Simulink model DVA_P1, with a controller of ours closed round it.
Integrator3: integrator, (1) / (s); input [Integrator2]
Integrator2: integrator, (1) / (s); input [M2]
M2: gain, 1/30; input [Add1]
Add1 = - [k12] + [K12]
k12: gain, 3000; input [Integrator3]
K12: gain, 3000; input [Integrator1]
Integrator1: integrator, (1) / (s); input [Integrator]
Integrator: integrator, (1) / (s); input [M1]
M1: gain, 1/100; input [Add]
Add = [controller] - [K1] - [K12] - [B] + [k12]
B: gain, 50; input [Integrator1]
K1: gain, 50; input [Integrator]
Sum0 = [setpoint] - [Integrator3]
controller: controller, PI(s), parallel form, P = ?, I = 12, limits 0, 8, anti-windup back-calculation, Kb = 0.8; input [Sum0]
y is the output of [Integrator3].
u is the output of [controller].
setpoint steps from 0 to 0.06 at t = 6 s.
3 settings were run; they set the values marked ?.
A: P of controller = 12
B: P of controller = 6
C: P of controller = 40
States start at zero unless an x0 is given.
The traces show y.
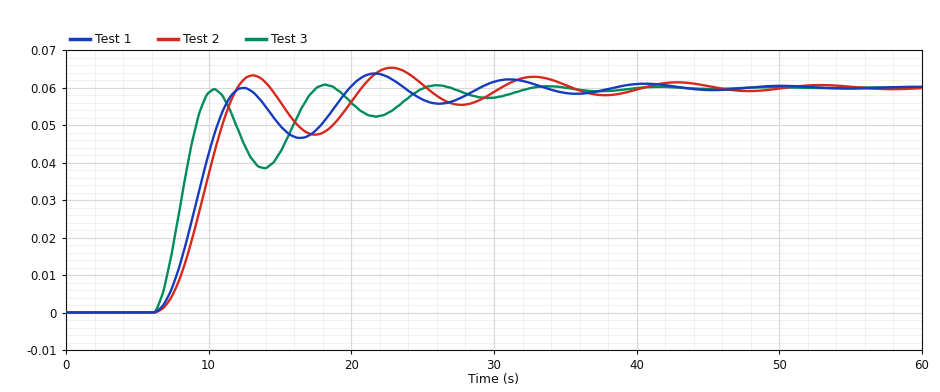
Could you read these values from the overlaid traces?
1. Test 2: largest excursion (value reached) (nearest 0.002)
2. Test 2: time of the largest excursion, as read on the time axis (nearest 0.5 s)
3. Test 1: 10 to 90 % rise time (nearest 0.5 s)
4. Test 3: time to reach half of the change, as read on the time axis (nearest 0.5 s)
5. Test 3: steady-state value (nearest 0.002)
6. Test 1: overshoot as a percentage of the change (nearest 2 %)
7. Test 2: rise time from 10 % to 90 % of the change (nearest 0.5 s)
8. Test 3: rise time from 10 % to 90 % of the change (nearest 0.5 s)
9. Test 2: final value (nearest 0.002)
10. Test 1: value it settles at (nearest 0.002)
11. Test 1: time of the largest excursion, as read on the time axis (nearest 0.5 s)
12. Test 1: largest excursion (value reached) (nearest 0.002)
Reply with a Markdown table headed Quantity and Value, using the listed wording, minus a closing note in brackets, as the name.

| Quantity | Value |
|---|---|
| Test 2: largest excursion (value reached) | 0.066 |
| Test 2: time of the largest excursion, as read on the time axis | 23.0 s |
| Test 1: 10 to 90 % rise time | 3.5 s |
| Test 3: time to reach half of the change, as read on the time axis | 8.0 s |
| Test 3: steady-state value | 0.060 |
| Test 1: overshoot as a percentage of the change | 6 % |
| Test 2: rise time from 10 % to 90 % of the change | 3.5 s |
| Test 3: rise time from 10 % to 90 % of the change | 2.5 s |
| Test 2: final value | 0.060 |
| Test 1: value it settles at | 0.060 |
| Test 1: time of the largest excursion, as read on the time axis | 21.5 s |
| Test 1: largest excursion (value reached) | 0.064 |
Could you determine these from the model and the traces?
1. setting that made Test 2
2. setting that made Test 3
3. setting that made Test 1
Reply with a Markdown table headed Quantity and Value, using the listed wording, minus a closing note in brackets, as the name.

| Quantity | Value |
|---|---|
| setting that made Test 2 | B |
| setting that made Test 3 | C |
| setting that made Test 1 | A |
